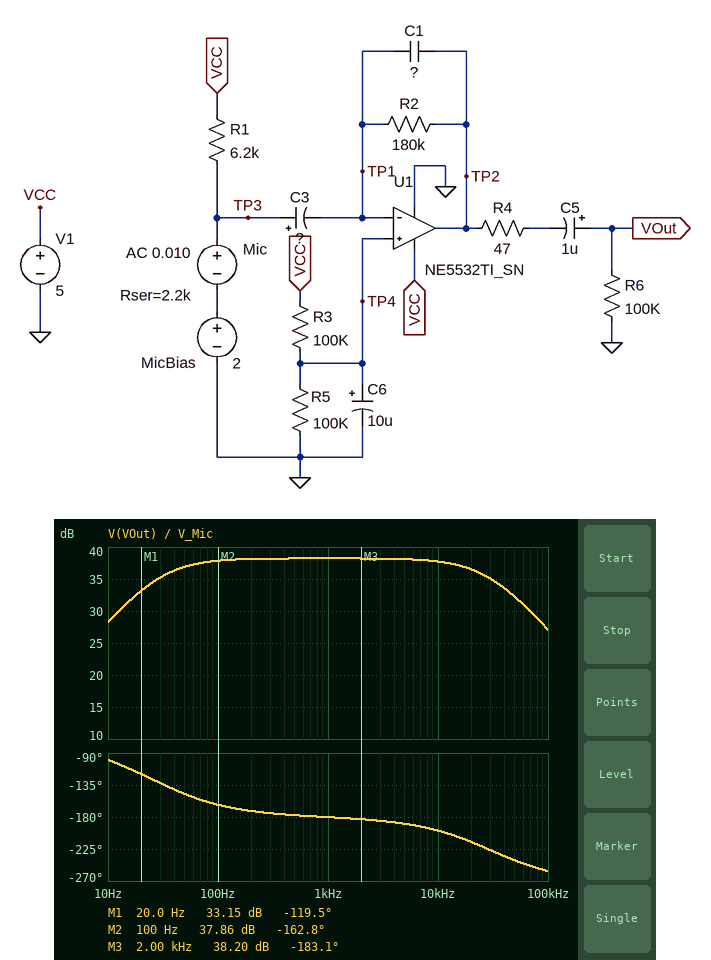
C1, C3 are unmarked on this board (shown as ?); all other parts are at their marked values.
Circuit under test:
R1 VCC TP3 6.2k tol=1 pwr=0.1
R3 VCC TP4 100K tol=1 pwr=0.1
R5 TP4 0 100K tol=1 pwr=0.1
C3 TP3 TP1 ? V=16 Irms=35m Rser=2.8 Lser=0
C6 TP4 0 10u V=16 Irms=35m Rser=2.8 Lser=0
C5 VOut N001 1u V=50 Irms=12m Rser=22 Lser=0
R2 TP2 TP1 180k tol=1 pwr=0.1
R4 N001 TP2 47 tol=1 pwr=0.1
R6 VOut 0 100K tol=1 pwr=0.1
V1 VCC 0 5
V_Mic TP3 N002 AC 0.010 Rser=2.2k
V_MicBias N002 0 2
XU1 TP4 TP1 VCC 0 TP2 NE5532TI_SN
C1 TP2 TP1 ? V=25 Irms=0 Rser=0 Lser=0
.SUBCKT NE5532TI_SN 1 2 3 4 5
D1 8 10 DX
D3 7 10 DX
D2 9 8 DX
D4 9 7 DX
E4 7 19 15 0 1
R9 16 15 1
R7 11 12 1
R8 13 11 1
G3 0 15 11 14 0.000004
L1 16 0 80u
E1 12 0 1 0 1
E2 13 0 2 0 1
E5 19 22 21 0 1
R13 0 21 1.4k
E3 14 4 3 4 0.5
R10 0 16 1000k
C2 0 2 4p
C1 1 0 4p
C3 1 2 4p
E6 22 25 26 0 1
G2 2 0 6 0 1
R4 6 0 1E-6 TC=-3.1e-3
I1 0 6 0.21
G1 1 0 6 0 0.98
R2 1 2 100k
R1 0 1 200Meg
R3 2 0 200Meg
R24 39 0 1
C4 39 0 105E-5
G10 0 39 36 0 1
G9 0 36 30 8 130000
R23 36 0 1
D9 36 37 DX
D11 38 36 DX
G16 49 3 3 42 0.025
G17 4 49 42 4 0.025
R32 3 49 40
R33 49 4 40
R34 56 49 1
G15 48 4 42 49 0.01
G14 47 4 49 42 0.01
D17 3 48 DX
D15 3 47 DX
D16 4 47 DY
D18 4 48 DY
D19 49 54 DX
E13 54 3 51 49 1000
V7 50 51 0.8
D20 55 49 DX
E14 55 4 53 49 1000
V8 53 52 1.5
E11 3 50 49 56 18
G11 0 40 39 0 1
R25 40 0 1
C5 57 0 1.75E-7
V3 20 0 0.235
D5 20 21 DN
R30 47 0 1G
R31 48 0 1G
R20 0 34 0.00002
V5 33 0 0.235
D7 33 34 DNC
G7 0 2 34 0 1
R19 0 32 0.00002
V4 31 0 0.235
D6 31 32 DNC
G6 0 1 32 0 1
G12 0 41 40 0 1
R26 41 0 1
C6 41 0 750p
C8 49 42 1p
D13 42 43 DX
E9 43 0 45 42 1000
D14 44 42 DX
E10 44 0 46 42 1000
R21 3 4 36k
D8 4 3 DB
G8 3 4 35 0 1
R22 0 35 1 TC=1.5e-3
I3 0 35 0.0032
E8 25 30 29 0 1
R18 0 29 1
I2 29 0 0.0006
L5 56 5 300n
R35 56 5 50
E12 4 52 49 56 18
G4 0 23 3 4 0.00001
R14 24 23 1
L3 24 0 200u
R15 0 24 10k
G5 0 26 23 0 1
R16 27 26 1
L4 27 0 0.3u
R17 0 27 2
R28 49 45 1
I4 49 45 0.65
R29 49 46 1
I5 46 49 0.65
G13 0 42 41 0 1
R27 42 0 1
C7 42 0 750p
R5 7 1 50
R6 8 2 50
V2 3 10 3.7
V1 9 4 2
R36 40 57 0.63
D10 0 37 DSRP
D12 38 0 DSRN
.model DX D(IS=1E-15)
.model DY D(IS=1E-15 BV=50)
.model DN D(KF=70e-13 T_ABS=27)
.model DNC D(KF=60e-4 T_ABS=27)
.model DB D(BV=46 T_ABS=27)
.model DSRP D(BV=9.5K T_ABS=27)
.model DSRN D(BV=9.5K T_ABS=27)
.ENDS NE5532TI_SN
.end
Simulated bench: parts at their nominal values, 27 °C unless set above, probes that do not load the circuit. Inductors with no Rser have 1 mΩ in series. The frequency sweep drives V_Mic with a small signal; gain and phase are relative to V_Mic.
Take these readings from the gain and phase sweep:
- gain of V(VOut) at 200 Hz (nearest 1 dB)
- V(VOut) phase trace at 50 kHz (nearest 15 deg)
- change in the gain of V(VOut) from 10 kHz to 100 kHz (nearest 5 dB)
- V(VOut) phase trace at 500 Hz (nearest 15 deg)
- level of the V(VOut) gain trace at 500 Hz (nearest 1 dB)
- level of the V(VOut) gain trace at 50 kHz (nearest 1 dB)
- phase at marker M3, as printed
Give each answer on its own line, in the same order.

38 dB
-240 deg
-10 dB
-180 deg
38 dB
32 dB
-183.1 deg
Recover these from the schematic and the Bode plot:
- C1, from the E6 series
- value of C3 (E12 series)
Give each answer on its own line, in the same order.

22 pF
3.3 µF
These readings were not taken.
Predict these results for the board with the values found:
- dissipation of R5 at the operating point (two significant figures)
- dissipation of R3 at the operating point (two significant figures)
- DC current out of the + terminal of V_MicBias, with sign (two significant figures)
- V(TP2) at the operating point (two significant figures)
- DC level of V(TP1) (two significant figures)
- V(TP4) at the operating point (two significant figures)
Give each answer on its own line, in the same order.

36 µW
96 µW
-360 µA
4.1 V
1.9 V
1.9 V
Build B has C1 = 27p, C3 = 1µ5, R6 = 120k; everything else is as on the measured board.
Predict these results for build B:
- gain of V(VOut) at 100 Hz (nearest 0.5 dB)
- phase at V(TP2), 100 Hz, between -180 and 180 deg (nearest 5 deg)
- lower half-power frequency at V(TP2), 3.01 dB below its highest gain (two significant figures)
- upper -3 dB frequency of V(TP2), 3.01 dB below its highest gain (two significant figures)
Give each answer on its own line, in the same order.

36.5 dB
-145 deg
65 Hz
25 kHz
